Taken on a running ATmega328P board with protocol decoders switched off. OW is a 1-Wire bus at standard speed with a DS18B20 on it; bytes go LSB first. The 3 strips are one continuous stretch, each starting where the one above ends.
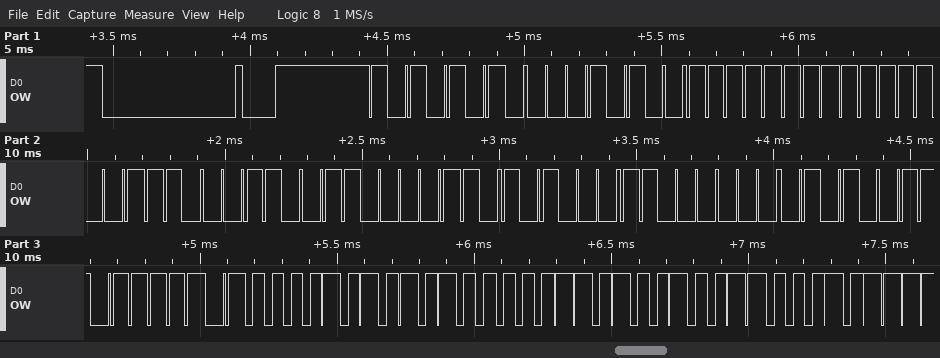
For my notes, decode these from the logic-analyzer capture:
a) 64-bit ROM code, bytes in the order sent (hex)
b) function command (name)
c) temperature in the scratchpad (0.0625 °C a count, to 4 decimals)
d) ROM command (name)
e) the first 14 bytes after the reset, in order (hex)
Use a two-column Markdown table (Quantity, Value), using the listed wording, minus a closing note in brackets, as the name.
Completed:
| Quantity | Value |
|---|---|
| 64-bit ROM code, bytes in the order sent | 28 FF 9F 63 86 15 03 CA |
| function command | Read Scratchpad |
| temperature in the scratchpad | 85.0000 °C |
| ROM command | Match ROM |
| the first 14 bytes after the reset, in order | 55 28 FF 9F 63 86 15 03 CA BE 50 05 4B 46 |
